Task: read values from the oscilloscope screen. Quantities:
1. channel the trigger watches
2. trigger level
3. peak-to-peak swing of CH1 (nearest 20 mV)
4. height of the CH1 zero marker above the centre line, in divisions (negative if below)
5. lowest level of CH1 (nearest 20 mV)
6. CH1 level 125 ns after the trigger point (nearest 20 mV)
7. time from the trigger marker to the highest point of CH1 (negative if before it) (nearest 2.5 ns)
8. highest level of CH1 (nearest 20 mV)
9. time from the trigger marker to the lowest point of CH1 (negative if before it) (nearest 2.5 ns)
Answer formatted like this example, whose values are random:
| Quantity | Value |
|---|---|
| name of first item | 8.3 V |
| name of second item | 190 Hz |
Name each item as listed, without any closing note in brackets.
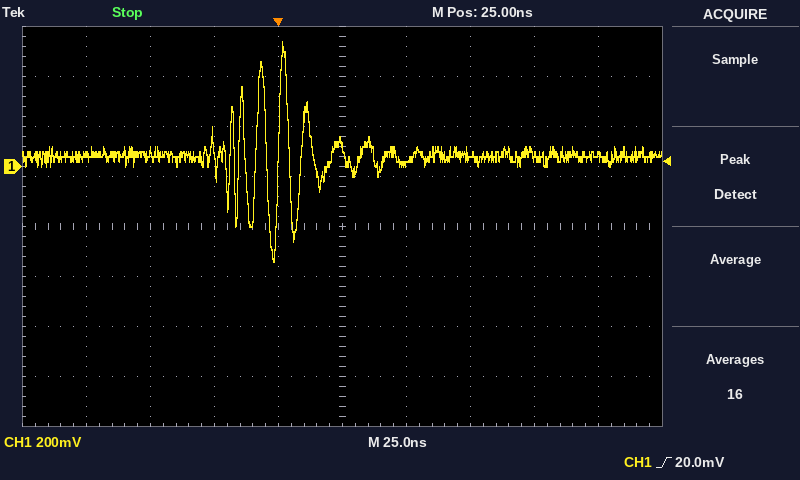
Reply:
| Quantity | Value |
|---|---|
| channel the trigger watches | CH1 |
| trigger level | 20.0 mV |
| peak-to-peak swing of CH1 | 880 mV |
| height of the CH1 zero marker above the centre line, in divisions | +1.2 div |
| lowest level of CH1 | -380 mV |
| CH1 level 125 ns after the trigger point | 40 mV |
| time from the trigger marker to the highest point of CH1 (negative if before it) | +2.5 ns |
| highest level of CH1 | 500 mV |
| time from the trigger marker to the lowest point of CH1 (negative if before it) | -2.5 ns |
